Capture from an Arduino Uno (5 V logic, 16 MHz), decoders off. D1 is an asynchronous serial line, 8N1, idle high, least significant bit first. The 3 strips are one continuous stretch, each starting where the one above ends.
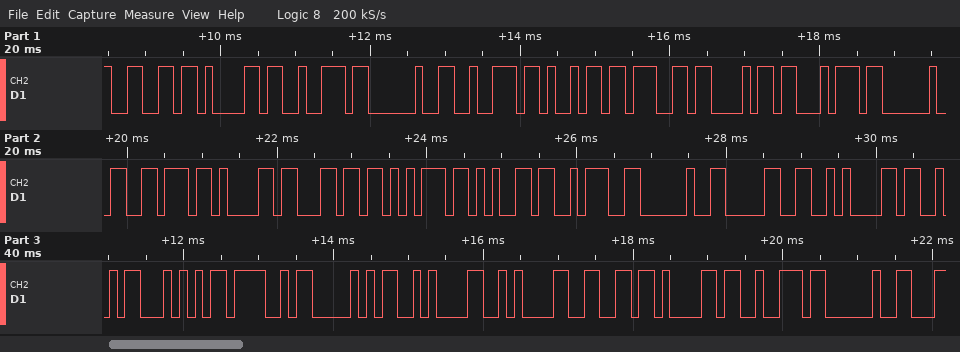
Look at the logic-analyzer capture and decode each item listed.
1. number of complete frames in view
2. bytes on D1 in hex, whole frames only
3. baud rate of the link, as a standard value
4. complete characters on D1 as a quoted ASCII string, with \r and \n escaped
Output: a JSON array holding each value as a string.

["29", "0x66 0x61 0x72 0x20 0x72 0x69 0x67 0x68 0x74 0x20 0x76 0x61 0x6C 0x75 0x65 0x3A 0x20 0x30 0x0A 0x53 0x54 0x4F 0x50 0x0A 0x0A 0x66 0x61 0x72 0x20", "9600 baud", "\"far right value: 0\\nSTOP\\n\\nfar \""]
